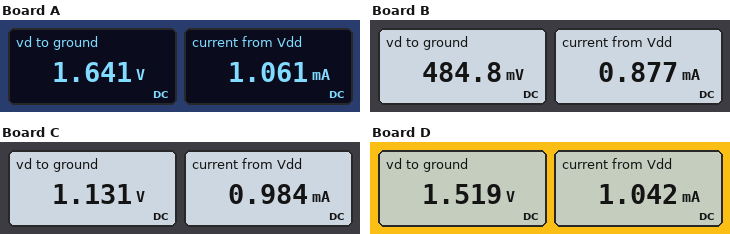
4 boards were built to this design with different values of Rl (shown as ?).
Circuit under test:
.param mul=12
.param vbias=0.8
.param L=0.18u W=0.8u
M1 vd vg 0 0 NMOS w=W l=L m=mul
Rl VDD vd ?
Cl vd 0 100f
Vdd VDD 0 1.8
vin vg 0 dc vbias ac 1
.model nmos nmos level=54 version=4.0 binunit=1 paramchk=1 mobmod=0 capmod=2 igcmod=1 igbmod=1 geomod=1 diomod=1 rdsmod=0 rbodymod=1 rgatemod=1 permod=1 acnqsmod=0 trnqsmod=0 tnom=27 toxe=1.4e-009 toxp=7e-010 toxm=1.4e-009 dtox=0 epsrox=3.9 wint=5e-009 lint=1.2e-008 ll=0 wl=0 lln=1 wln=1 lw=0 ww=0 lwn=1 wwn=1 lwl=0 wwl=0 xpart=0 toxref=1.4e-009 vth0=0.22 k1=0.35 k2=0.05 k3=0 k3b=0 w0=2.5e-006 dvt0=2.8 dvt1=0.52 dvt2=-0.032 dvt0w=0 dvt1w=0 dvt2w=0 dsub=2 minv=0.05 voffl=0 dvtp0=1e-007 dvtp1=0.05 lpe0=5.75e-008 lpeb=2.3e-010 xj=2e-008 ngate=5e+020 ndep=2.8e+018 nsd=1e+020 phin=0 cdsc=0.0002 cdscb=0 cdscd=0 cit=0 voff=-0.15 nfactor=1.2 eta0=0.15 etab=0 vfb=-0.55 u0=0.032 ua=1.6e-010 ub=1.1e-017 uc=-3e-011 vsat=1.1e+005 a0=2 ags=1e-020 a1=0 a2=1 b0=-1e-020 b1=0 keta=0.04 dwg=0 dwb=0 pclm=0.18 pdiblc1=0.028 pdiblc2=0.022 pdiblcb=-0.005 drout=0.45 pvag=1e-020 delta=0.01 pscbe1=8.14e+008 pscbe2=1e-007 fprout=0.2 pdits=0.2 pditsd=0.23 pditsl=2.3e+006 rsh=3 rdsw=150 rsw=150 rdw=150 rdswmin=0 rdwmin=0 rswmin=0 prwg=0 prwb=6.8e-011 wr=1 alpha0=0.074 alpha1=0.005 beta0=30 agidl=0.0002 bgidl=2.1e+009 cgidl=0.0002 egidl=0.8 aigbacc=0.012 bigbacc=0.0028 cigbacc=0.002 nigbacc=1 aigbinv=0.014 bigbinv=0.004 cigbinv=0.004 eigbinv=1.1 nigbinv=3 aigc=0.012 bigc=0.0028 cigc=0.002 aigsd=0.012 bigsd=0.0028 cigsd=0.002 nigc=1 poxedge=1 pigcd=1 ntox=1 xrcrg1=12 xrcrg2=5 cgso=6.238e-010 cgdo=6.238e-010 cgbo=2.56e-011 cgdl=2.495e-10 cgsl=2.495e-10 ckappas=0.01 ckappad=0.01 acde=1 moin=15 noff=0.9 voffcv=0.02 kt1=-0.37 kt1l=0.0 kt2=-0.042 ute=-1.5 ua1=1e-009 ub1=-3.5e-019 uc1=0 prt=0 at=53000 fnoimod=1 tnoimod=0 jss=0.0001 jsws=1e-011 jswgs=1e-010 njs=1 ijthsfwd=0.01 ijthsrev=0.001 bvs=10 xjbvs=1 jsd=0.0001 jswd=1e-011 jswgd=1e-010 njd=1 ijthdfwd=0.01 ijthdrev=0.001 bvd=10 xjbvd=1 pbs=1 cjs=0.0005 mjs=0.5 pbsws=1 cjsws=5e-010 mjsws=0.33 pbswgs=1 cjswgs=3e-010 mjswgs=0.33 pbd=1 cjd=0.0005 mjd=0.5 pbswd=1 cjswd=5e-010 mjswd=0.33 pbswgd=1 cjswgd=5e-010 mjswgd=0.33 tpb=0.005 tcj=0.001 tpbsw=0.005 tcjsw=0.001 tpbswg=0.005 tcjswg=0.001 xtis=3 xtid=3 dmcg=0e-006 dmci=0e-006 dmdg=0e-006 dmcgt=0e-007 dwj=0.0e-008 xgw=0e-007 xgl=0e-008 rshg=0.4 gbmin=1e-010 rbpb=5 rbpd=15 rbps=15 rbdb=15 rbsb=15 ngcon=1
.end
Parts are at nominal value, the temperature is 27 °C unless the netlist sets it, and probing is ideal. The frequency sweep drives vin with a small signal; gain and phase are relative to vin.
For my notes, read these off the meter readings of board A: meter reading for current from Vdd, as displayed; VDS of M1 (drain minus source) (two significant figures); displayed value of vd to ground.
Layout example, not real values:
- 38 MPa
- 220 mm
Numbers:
- 1.061 mA
- 1.6 V
- 1.641 V
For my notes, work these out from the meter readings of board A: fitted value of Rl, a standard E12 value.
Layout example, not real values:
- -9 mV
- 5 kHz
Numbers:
- 150 Ω
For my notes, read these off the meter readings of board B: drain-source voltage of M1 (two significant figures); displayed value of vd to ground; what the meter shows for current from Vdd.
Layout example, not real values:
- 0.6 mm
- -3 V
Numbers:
- 480 mV
- 484.8 mV
- 0.877 mA
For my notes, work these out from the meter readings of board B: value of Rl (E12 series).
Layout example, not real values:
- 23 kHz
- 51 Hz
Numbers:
- 1.5 kΩ
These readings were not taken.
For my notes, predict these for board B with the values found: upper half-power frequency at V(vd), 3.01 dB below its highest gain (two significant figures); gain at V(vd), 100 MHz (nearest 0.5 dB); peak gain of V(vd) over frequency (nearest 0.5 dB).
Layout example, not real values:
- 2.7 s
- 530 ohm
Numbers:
- 1.3 GHz
- 6.5 dB
- 6.5 dB
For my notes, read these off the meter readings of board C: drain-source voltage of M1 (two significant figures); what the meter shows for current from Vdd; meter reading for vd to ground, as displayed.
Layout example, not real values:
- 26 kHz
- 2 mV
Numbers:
- 1.1 V
- 0.984 mA
- 1.131 V
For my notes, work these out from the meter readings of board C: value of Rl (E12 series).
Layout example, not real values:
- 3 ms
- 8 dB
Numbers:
- 680 Ω
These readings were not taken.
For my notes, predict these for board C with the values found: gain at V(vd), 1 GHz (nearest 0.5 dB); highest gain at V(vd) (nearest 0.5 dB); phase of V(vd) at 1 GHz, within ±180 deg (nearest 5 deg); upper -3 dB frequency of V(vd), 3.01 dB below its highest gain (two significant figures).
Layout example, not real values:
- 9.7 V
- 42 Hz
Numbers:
- 1.5 dB
- 2.5 dB
- 155 deg
- 2.4 GHz
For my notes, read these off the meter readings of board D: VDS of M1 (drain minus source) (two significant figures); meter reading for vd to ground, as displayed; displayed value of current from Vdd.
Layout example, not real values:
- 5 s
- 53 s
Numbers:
- 1.5 V
- 1.519 V
- 1.042 mA
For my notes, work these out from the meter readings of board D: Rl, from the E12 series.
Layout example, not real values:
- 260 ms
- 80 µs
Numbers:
- 270 Ω
